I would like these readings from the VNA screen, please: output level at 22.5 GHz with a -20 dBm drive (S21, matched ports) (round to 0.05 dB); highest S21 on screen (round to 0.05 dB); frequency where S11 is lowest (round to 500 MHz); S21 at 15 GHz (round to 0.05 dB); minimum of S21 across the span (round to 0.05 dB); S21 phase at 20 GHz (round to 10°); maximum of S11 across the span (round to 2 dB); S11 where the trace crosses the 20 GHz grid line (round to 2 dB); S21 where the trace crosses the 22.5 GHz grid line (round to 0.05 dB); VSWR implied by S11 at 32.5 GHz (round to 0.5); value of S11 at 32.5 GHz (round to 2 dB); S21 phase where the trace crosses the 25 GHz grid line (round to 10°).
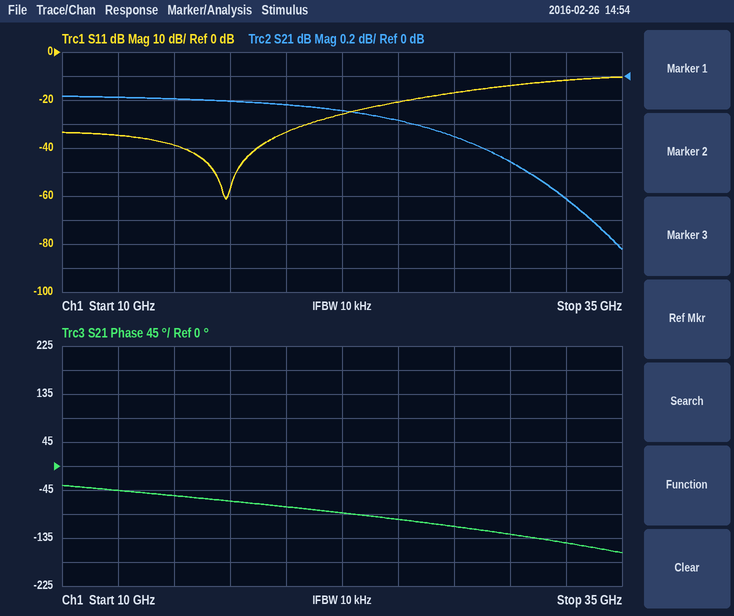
-20.30 dBm
-0.15 dB
17.5 GHz
-0.20 dB
-1.45 dB
-80°
-10 dB
-34 dB
-0.30 dB
1.5
-12 dB
-100°
